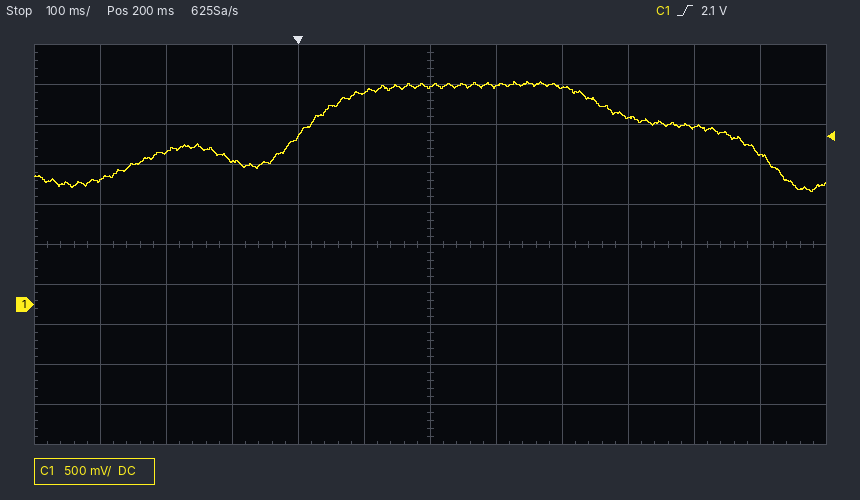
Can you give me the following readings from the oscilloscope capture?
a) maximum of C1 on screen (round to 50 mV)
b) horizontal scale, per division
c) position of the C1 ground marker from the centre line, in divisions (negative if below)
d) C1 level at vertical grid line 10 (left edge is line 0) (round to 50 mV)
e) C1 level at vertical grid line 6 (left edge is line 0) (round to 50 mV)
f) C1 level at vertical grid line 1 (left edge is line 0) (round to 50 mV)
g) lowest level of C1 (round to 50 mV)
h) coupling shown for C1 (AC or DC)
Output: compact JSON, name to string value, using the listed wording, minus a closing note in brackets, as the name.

{"maximum of C1 on screen": "2.80 V", "horizontal scale, per division": "100 ms", "position of the C1 ground marker from the centre line, in divisions": "-1.5 div", "C1 level at vertical grid line 10 (left edge is line 0)": "2.20 V", "C1 level at vertical grid line 6 (left edge is line 0)": "2.70 V", "C1 level at vertical grid line 1 (left edge is line 0)": "1.55 V", "lowest level of C1": "1.40 V", "coupling shown for C1": "DC"}
